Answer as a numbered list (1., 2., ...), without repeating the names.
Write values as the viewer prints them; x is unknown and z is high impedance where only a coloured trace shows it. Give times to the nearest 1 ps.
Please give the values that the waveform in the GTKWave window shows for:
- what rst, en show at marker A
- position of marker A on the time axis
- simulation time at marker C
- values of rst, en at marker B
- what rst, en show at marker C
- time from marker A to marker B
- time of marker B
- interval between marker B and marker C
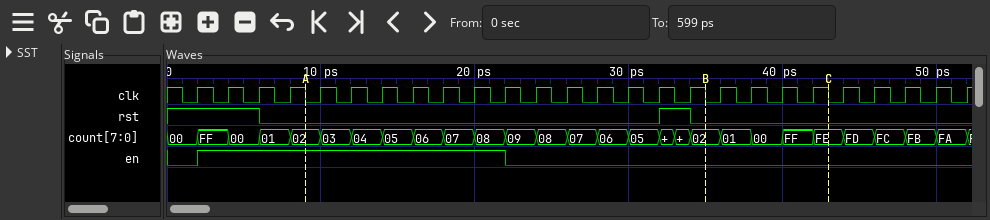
1. rst=0, en=1
2. 9 ps
3. 43 ps
4. rst=0, en=0
5. rst=0, en=0
6. 26 ps
7. 35 ps
8. 8 ps
